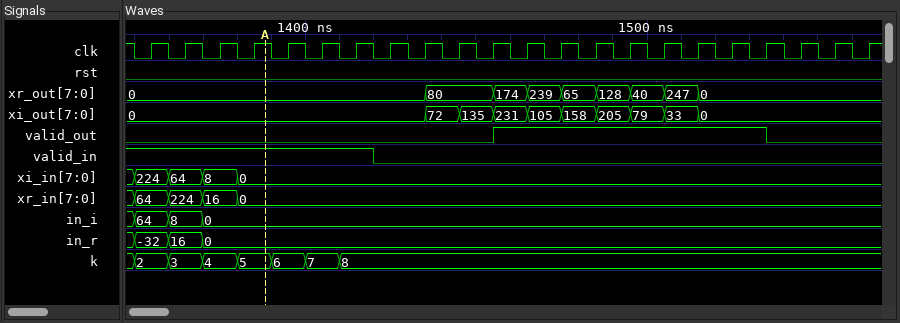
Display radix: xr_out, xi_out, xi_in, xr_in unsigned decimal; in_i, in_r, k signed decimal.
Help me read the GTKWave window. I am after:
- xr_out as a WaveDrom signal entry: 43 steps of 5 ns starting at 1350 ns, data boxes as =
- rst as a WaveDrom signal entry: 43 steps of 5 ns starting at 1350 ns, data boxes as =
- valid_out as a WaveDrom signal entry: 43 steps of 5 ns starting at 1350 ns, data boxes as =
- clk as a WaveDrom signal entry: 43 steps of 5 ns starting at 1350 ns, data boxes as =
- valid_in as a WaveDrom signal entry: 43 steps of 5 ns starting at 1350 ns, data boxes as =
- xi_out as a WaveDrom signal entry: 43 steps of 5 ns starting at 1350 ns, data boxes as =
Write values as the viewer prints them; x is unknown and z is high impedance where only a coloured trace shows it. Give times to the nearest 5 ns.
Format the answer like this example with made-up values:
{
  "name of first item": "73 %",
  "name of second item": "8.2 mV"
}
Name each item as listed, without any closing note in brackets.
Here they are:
{
  "xr_out as a WaveDrom signal entry: 43 steps of 5 ns starting at 1350 ns, data boxes as =": "{name: 'xr_out', wave: '=................=...=.=.=.=.=.=.=.........', data: '0 80 174 239 65 128 40 247 0'}",
  "rst as a WaveDrom signal entry: 43 steps of 5 ns starting at 1350 ns, data boxes as =": "{name: 'rst', wave: '0..........................................'}",
  "valid_out as a WaveDrom signal entry: 43 steps of 5 ns starting at 1350 ns, data boxes as =": "{name: 'valid_out', wave: '0....................1...............0.....'}",
  "clk as a WaveDrom signal entry: 43 steps of 5 ns starting at 1350 ns, data boxes as =": "{name: 'clk', wave: '0101010101010101010101010101010101010101010'}",
  "valid_in as a WaveDrom signal entry: 43 steps of 5 ns starting at 1350 ns, data boxes as =": "{name: 'valid_in', wave: '1.............0............................'}",
  "xi_out as a WaveDrom signal entry: 43 steps of 5 ns starting at 1350 ns, data boxes as =": "{name: 'xi_out', wave: '=................=.=.=.=.=.=.=.=.=.........', data: '0 72 135 231 105 158 205 79 33 0'}"
}
